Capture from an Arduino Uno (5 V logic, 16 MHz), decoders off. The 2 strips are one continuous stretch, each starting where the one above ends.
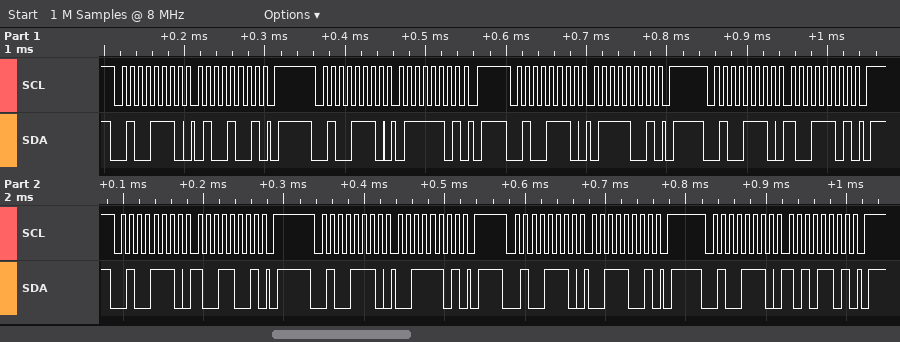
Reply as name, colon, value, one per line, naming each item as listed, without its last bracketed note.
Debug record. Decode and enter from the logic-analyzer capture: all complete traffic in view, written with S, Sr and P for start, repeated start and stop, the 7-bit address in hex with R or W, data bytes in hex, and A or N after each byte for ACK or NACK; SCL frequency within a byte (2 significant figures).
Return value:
all complete traffic in view, written with S, Sr and P for start, repeated start and stop, the 7-bit address in hex with R or W, data bytes in hex, and A or N after each byte for ACK or NACK: S 27W A 49 A P S 27W A 7D A P S 27W A 79 A P S 27W A 9D A P S 27W A 99 A P S 27W A 3D A P S 27W A 39 A P S 27W A AD A P
SCL frequency within a byte: 100 kHz
